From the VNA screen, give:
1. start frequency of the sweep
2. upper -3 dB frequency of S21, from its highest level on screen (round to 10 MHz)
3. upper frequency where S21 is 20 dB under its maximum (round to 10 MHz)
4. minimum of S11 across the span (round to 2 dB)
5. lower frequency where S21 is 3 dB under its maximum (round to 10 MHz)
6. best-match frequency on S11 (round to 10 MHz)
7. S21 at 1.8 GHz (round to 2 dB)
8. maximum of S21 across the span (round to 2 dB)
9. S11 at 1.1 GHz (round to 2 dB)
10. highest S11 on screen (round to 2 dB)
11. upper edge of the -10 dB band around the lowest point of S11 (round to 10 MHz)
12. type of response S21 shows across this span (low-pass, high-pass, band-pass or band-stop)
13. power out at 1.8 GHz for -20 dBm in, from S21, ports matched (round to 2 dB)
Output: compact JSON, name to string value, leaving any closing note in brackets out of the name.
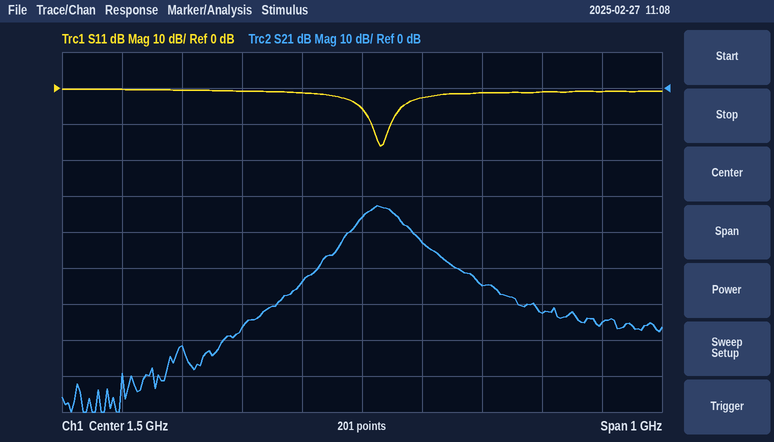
{"start frequency of the sweep": "1 GHz", "upper -3 dB frequency of S21, from its highest level on screen": "1.56 GHz", "upper frequency where S21 is 20 dB under its maximum": "1.69 GHz", "minimum of S11 across the span": "-16 dB", "lower frequency where S21 is 3 dB under its maximum": "1.50 GHz", "best-match frequency on S11": "1.53 GHz", "S21 at 1.8 GHz": "-62 dB", "maximum of S21 across the span": "-32 dB", "S11 at 1.1 GHz": "0 dB", "highest S11 on screen": "0 dB", "upper edge of the -10 dB band around the lowest point of S11": "1.55 GHz", "type of response S21 shows across this span": "band-pass", "power out at 1.8 GHz for -20 dBm in, from S21, ports matched": "-82 dBm"}
